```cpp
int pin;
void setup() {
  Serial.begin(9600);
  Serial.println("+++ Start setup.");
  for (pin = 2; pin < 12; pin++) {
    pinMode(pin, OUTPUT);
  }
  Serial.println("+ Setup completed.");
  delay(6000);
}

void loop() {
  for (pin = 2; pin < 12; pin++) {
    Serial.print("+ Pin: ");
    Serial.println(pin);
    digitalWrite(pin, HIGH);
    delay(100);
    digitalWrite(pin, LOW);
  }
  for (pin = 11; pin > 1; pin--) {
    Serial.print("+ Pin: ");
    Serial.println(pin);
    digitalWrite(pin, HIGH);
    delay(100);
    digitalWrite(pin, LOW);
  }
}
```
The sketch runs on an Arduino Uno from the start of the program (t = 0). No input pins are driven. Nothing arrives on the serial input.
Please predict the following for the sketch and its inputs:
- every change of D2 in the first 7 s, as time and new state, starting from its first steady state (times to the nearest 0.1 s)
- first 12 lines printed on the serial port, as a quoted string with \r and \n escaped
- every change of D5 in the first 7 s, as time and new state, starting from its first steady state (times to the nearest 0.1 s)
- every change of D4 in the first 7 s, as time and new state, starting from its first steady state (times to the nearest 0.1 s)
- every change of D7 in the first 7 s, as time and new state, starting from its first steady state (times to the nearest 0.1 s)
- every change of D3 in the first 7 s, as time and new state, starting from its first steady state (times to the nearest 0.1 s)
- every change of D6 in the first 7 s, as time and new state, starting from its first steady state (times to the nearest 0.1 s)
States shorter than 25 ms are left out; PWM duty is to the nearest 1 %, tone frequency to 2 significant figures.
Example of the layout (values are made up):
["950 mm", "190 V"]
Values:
["0 s low; 6 s high; 6.1 s low", "\"+++ Start setup.\\r\\n+ Setup completed.\\r\\n+ Pin: 2\\r\\n+ Pin: 3\\r\\n+ Pin: 4\\r\\n+ Pin: 5\\r\\n+ Pin: 6\\r\\n+ Pin: 7\\r\\n+ Pin: 8\\r\\n+ Pin: 9\\r\\n+ Pin: 10\\r\\n+ Pin: 11\\r\\n\"", "0 s low; 6.3 s high; 6.4 s low", "0 s low; 6.2 s high; 6.3 s low", "0 s low; 6.5 s high; 6.6 s low", "0 s low; 6.1 s high; 6.2 s low", "0 s low; 6.4 s high; 6.5 s low"]
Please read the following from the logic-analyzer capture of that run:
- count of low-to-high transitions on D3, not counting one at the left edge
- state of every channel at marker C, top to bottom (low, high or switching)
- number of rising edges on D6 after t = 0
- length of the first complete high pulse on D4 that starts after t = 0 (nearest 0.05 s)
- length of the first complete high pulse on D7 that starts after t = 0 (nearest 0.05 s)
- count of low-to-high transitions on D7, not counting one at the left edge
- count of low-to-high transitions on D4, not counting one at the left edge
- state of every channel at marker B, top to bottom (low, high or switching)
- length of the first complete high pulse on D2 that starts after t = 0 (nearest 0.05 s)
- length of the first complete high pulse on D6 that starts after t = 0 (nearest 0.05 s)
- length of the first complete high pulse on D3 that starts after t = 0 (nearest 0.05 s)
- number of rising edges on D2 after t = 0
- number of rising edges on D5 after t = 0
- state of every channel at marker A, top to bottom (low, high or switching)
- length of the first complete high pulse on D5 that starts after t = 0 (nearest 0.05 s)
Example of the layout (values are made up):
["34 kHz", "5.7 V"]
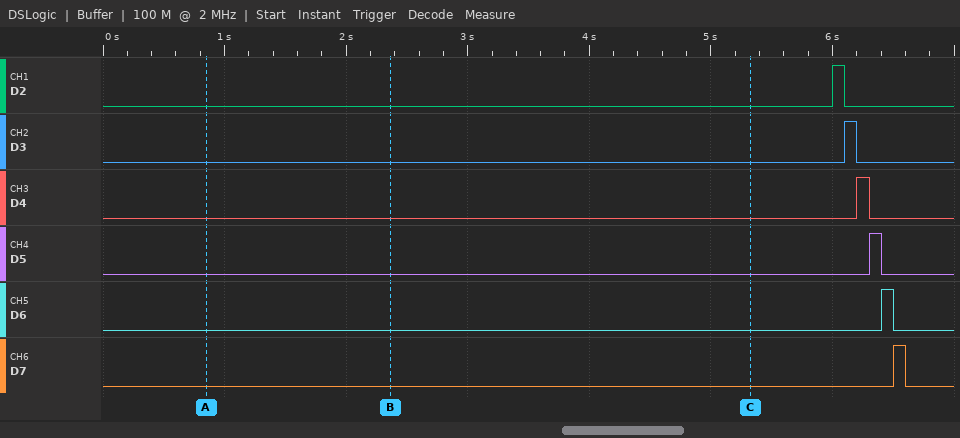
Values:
["1", "D2 low, D3 low, D4 low, D5 low, D6 low, D7 low", "1", "0.10 s", "0.10 s", "1", "1", "D2 low, D3 low, D4 low, D5 low, D6 low, D7 low", "0.10 s", "0.10 s", "0.10 s", "1", "1", "D2 low, D3 low, D4 low, D5 low, D6 low, D7 low", "0.10 s"]
